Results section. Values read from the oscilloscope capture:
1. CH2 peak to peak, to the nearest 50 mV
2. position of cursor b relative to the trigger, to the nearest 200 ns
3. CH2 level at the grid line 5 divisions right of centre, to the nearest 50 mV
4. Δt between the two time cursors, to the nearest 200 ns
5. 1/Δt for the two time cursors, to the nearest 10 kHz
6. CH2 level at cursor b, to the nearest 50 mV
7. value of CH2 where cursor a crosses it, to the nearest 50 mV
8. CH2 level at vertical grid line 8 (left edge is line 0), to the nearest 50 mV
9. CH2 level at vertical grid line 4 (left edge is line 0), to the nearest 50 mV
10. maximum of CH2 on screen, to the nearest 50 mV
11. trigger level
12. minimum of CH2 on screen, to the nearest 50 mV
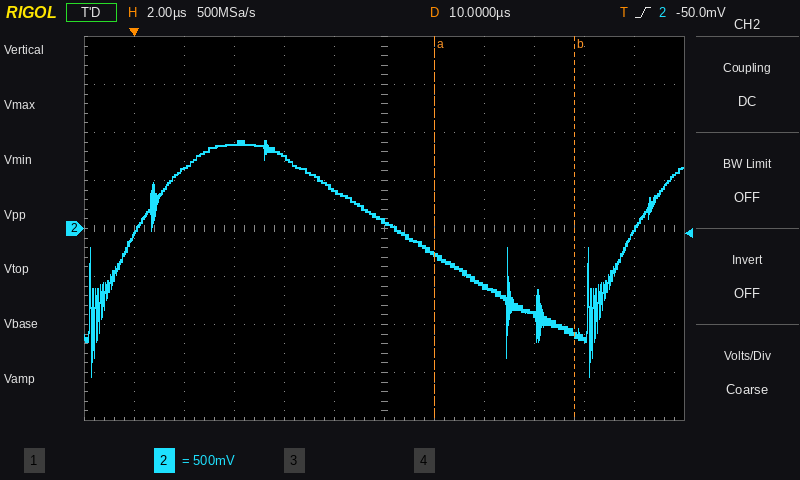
2.45 V
+17.6 µs
0 mV
5.6 µs
180 kHz
-1.10 V
-300 mV
-600 mV
750 mV
900 mV
-50.0 mV
-1.55 V
